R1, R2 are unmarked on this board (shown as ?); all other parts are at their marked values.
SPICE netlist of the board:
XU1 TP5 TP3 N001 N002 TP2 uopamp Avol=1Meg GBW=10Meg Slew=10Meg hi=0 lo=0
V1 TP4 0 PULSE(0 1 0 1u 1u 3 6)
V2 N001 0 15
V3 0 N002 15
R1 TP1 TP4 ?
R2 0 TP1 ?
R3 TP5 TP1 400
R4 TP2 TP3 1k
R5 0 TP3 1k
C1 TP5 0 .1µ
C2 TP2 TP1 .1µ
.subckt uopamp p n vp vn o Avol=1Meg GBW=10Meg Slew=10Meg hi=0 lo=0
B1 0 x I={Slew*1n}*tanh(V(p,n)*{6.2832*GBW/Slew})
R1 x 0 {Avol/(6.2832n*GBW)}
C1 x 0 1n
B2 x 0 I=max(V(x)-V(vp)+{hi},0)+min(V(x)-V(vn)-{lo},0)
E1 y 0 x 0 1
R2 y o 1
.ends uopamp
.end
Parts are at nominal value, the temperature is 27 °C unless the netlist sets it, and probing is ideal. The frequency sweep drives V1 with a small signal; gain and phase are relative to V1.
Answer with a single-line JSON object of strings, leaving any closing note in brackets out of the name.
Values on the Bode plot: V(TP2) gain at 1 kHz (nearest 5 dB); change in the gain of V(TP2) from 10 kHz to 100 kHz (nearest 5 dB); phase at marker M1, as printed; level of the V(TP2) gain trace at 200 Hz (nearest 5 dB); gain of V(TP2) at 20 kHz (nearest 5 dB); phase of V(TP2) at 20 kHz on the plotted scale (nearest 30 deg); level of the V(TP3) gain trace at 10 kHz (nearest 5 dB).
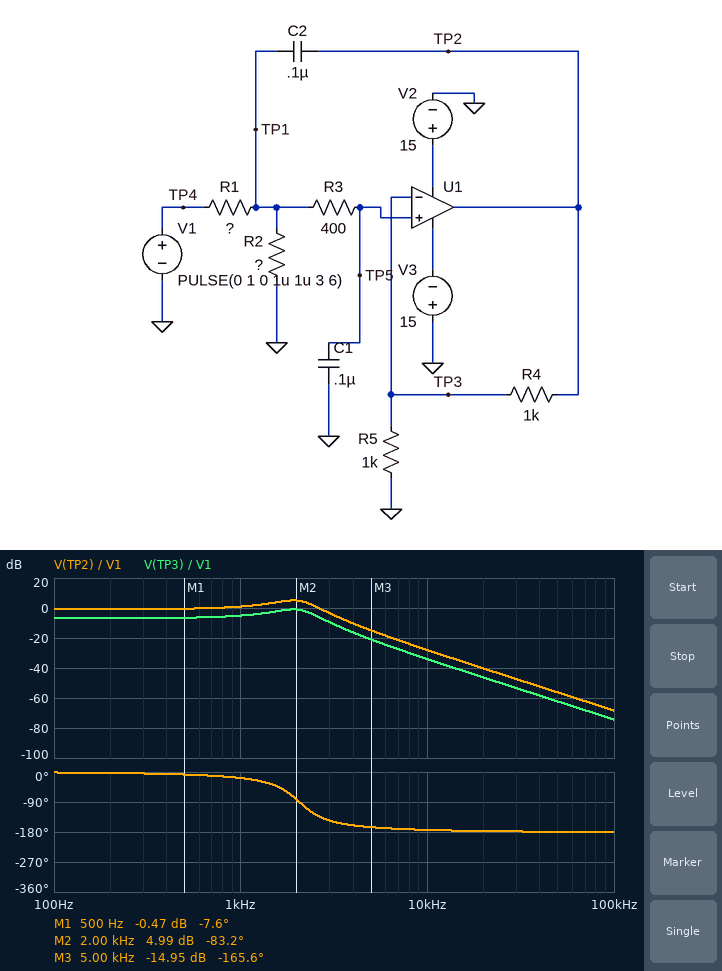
{"V(TP2) gain at 1 kHz": "0 dB", "change in the gain of V(TP2) from 10 kHz to 100 kHz": "-40 dB", "phase at marker M1, as printed": "-7.6 deg", "level of the V(TP2) gain trace at 200 Hz": "0 dB", "gain of V(TP2) at 20 kHz": "-40 dB", "phase of V(TP2) at 20 kHz on the plotted scale": "-180 deg", "level of the V(TP3) gain trace at 10 kHz": "-35 dB"}
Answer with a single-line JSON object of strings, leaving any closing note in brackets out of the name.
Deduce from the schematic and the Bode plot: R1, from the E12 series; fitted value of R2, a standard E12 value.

{"R1, from the E12 series": "3.3 kΩ", "fitted value of R2, a standard E12 value": "2.7 kΩ"}
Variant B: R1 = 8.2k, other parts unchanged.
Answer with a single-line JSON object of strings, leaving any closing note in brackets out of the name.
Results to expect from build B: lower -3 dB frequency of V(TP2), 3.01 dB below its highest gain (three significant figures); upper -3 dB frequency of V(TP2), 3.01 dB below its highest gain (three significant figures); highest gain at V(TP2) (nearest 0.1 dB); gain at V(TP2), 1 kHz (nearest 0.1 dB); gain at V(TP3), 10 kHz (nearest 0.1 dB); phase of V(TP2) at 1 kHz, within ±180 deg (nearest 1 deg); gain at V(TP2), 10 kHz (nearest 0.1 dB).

{"lower -3 dB frequency of V(TP2), 3.01 dB below its highest gain": "1.21 kHz", "upper -3 dB frequency of V(TP2), 3.01 dB below its highest gain": "2.04 kHz", "highest gain at V(TP2)": "1.2 dB", "gain at V(TP2), 1 kHz": "-3.3 dB", "gain at V(TP3), 10 kHz": "-42.0 dB", "phase of V(TP2) at 1 kHz, within ±180 deg": "-20 deg", "gain at V(TP2), 10 kHz": "-36.0 dB"}
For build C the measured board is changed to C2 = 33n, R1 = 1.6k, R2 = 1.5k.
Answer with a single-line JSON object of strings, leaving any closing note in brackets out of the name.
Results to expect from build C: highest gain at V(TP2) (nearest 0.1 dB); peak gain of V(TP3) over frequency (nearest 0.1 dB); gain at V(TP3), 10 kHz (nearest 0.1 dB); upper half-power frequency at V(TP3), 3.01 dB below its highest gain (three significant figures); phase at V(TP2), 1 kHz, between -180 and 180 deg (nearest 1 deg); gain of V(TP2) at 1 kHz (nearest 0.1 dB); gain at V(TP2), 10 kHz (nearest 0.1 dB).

{"highest gain at V(TP2)": "-0.3 dB", "peak gain of V(TP3) over frequency": "-6.3 dB", "gain at V(TP3), 10 kHz": "-22.6 dB", "upper half-power frequency at V(TP3), 3.01 dB below its highest gain": "1.97 kHz", "phase at V(TP2), 1 kHz, between -180 and 180 deg": "-31 deg", "gain of V(TP2) at 1 kHz": "-1.3 dB", "gain at V(TP2), 10 kHz": "-16.6 dB"}
